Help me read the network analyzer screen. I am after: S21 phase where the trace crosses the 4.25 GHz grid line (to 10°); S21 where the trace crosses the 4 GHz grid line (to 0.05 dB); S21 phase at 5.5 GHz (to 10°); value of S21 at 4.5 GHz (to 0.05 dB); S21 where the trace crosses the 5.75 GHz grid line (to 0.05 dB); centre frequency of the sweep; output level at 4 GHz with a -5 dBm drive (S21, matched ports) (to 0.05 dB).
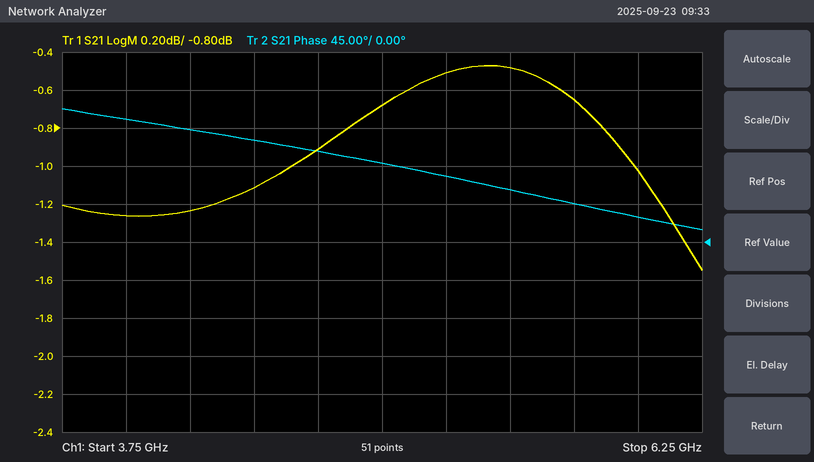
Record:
130°
-1.25 dB
60°
-1.10 dB
-0.65 dB
5 GHz
-6.25 dBm
